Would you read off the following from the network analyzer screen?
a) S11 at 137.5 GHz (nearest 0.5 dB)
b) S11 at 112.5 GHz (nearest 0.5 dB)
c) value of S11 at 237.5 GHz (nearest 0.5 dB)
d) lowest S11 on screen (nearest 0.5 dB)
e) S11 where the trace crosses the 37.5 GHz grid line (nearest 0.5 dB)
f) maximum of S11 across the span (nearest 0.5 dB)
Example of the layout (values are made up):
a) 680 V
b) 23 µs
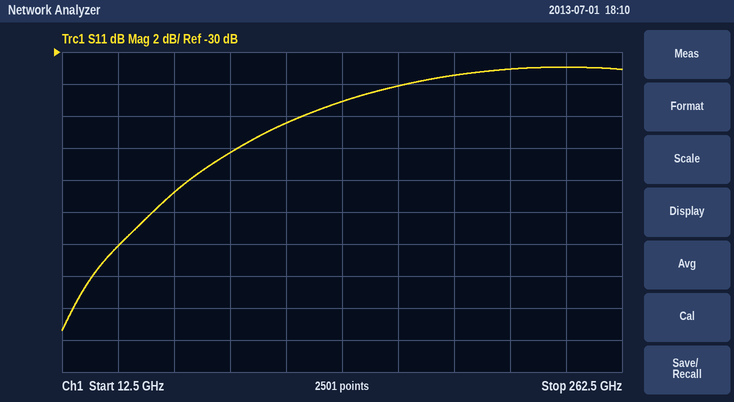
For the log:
a) -33.0 dB
b) -34.5 dB
c) -31.0 dB
d) -47.5 dB
e) -42.0 dB
f) -31.0 dB
